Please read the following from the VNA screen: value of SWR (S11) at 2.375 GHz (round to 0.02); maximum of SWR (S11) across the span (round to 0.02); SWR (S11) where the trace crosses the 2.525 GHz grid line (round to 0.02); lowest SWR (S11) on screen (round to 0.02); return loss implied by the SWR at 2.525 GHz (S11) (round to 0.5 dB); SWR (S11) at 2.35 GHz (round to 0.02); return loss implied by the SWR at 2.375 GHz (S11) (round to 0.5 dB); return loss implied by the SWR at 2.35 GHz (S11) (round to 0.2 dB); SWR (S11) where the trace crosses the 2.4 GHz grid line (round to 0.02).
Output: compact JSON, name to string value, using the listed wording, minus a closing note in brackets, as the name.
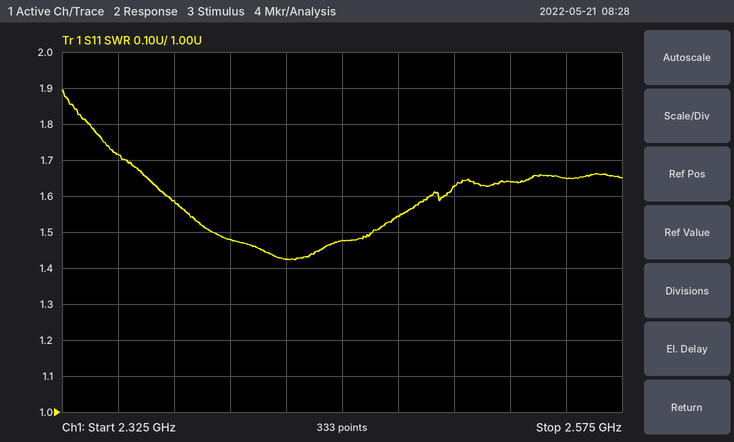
{"value of SWR (S11) at 2.375 GHz": "1.58", "maximum of SWR (S11) across the span": "1.90", "SWR (S11) where the trace crosses the 2.525 GHz grid line": "1.64", "lowest SWR (S11) on screen": "1.42", "return loss implied by the SWR at 2.525 GHz (S11)": "12.5 dB", "SWR (S11) at 2.35 GHz": "1.72", "return loss implied by the SWR at 2.375 GHz (S11)": "13.0 dB", "return loss implied by the SWR at 2.35 GHz (S11)": "11.6 dB", "SWR (S11) where the trace crosses the 2.4 GHz grid line": "1.48"}
